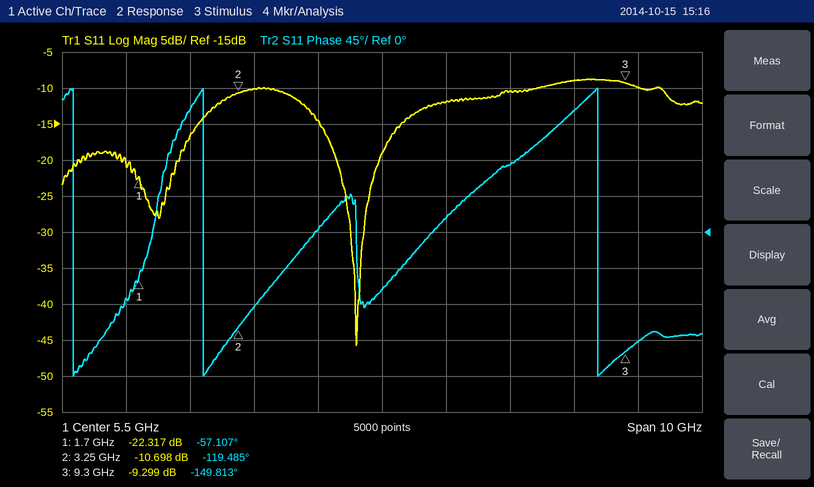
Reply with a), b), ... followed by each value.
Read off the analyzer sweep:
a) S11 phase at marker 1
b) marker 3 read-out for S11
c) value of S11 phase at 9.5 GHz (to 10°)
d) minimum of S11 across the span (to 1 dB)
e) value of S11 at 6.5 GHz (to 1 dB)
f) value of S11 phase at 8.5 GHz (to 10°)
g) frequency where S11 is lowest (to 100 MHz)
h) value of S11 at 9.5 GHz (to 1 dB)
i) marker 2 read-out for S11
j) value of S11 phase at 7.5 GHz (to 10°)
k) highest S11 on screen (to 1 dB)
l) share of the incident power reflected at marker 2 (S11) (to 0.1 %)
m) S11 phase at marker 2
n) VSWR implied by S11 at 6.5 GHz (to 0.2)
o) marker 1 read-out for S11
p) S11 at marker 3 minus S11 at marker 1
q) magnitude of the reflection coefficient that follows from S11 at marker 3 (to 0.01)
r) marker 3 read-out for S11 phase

a) -57.107°
b) -9.299 dB
c) -140°
d) -46 dB
e) -12 dB
f) 150°
g) 5.1 GHz
h) -10 dB
i) -10.698 dB
j) 80°
k) -9 dB
l) 8.5 %
m) -119.485°
n) 1.6
o) -22.317 dB
p) 13.018 dB
q) 0.34
r) -149.813°
